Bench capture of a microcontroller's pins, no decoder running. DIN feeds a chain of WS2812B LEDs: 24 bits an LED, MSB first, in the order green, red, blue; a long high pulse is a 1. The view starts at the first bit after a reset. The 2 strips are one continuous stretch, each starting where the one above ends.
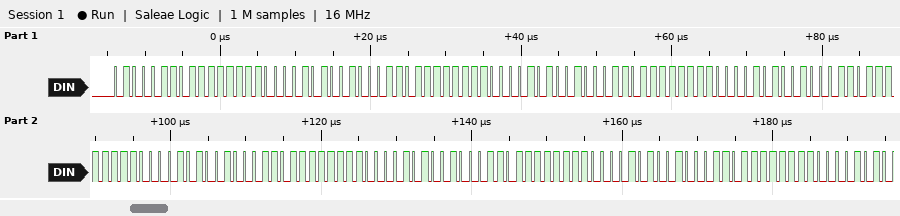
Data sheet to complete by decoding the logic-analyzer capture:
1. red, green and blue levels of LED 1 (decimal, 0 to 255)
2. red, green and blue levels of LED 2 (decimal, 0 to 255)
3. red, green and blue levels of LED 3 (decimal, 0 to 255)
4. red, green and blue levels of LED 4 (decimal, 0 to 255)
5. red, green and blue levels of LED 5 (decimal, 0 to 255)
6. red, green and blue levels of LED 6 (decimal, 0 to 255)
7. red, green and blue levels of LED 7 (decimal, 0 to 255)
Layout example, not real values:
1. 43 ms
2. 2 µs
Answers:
1. 255, 70, 10
2. 255, 70, 10
3. 255, 70, 10
4. 255, 70, 10
5. 255, 70, 10
6. 255, 70, 10
7. 255, 70, 10
